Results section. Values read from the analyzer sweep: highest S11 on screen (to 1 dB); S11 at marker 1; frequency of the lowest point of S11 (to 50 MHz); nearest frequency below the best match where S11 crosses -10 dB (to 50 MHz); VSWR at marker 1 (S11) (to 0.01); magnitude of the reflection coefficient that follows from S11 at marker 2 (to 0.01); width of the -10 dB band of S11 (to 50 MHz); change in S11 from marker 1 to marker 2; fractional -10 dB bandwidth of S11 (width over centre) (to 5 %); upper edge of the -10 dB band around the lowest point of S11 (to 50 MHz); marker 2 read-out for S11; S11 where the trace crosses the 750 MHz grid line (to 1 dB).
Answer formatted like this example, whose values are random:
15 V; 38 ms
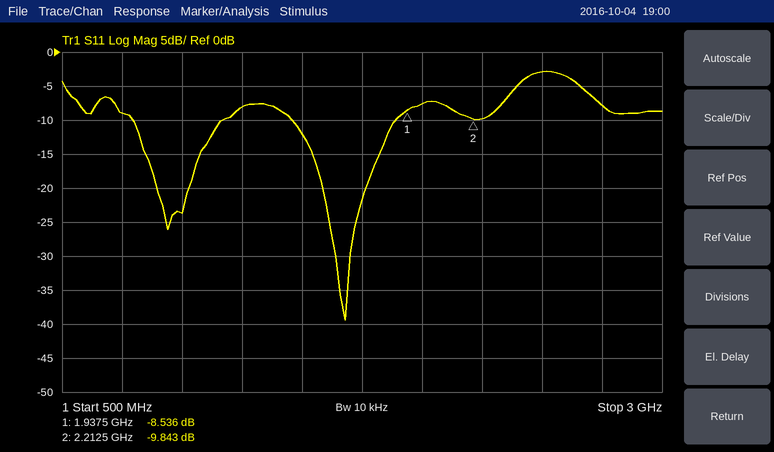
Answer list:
-3 dB; -8.536 dB; 1.70 GHz; 1.45 GHz; 2.20; 0.32; 450 MHz; -1.307 dB; 25 %; 1.90 GHz; -9.843 dB; -9 dB
